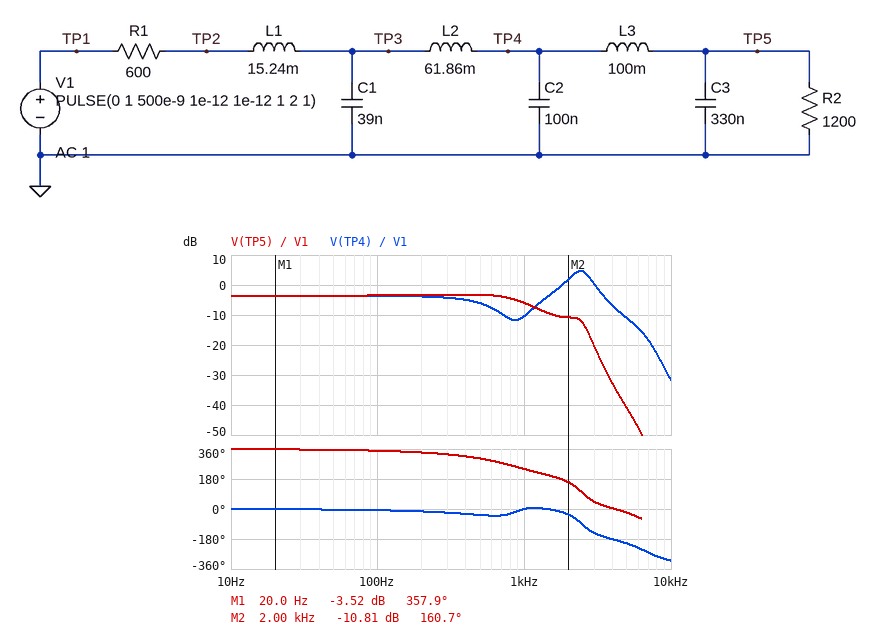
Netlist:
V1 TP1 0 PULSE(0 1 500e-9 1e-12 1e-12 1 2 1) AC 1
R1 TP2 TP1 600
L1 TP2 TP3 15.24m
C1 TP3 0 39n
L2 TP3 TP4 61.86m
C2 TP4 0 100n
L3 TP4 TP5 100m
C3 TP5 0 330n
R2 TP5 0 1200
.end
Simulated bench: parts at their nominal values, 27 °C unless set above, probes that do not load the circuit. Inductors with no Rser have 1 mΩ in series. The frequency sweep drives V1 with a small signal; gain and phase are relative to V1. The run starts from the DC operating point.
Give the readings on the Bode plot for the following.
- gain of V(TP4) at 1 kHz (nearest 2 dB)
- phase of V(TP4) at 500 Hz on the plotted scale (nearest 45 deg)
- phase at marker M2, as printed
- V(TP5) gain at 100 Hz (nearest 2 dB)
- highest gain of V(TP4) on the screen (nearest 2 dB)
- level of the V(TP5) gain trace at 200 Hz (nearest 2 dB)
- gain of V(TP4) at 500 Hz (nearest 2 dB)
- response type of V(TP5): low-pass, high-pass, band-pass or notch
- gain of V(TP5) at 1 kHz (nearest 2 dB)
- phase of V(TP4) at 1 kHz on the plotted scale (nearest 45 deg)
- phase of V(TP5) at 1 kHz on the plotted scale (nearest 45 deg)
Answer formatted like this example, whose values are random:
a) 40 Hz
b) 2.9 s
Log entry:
a) -10 dB
b) -45 deg
c) 160.7 deg
d) -4 dB
e) 4 dB
f) -4 dB
g) -6 dB
h) low-pass
i) -6 dB
j) 0 deg
k) 225 deg
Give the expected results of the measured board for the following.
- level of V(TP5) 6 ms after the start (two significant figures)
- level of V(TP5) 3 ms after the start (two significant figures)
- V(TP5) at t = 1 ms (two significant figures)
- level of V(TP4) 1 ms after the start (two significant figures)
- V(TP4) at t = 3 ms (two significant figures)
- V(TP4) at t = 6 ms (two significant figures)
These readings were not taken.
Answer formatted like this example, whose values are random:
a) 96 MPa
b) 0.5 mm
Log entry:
a) 670 mV
b) 670 mV
c) 690 mV
d) 720 mV
e) 670 mV
f) 670 mV
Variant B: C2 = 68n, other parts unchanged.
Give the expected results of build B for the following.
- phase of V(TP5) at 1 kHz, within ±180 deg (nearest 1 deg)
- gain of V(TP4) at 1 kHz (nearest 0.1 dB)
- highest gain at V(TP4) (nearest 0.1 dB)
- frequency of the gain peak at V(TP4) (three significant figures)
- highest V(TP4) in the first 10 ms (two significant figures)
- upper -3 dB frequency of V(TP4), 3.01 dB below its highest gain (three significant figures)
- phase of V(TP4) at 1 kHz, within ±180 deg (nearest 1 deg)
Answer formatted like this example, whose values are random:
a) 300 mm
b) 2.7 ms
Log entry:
a) -118 deg
b) -10.6 dB
c) 5.8 dB
d) 2.96 kHz
e) 830 mV
f) 3.48 kHz
g) 2 deg
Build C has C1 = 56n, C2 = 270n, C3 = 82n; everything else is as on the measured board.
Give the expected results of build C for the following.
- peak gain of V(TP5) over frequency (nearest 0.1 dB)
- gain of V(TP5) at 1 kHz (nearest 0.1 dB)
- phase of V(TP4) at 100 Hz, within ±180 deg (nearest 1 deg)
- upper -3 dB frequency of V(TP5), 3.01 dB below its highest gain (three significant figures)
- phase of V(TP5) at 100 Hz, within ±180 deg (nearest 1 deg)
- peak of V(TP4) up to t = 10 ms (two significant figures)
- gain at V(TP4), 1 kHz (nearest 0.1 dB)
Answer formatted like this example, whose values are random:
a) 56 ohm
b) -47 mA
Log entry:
a) -3.4 dB
b) -3.6 dB
c) -6 deg
d) 1.98 kHz
e) -9 deg
f) 680 mV
g) -4.9 dB
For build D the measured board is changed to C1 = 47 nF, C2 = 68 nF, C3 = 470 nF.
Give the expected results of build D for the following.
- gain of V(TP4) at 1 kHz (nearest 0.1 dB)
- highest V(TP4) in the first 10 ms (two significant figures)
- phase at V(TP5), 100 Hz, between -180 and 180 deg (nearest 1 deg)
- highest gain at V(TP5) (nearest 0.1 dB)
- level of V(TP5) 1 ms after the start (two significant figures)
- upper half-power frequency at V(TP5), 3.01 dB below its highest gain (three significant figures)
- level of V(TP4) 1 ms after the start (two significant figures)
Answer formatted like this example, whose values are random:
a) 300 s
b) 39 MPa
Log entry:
a) -8.7 dB
b) 840 mV
c) -12 deg
d) -3.4 dB
e) 710 mV
f) 808 Hz
g) 660 mV
